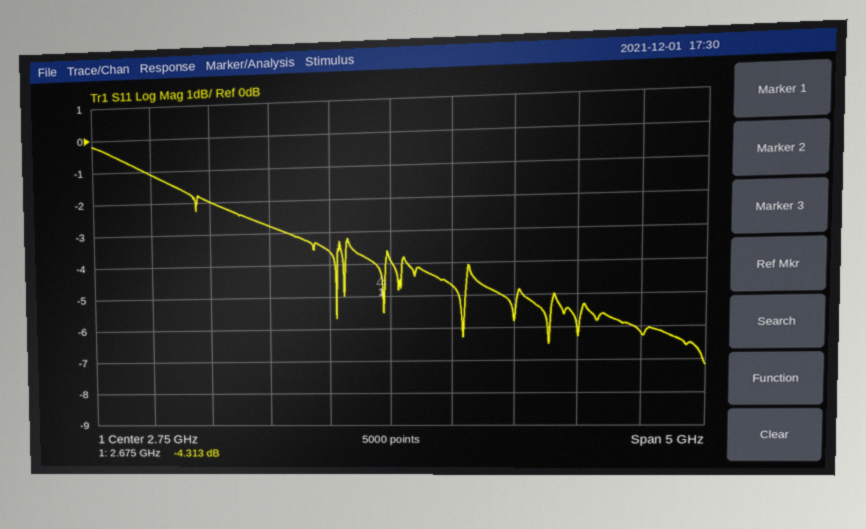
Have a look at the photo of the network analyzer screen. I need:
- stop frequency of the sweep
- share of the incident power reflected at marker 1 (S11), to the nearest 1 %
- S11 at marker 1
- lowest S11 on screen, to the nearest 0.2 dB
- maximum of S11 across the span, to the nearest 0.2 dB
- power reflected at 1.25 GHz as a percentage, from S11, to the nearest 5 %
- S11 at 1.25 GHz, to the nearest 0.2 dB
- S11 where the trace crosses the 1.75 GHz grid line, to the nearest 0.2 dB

5.25 GHz
37 %
-4.313 dB
-7.2 dB
-0.2 dB
65 %
-2.0 dB
-2.8 dB
